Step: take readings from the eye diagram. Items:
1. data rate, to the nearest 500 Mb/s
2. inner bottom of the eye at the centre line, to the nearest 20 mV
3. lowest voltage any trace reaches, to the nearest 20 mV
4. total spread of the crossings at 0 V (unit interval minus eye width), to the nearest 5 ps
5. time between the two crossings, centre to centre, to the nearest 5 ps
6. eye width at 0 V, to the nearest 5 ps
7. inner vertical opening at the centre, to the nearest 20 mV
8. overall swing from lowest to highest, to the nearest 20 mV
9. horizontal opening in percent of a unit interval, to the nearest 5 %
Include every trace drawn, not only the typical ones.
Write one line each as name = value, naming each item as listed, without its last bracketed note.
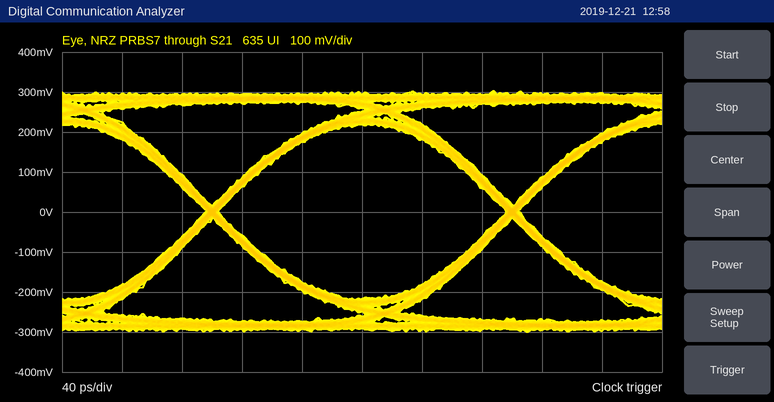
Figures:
data rate, to the nearest 500 Mb/s = 5.0 Gb/s
inner bottom of the eye at the centre line, to the nearest 20 mV = -220 mV
lowest voltage any trace reaches, to the nearest 20 mV = -300 mV
total spread of the crossings at 0 V (unit interval minus eye width), to the nearest 5 ps = 10 ps
time between the two crossings, centre to centre, to the nearest 5 ps = 200 ps
eye width at 0 V, to the nearest 5 ps = 190 ps
inner vertical opening at the centre, to the nearest 20 mV = 440 mV
overall swing from lowest to highest, to the nearest 20 mV = 600 mV
horizontal opening in percent of a unit interval, to the nearest 5 % = 95 %
